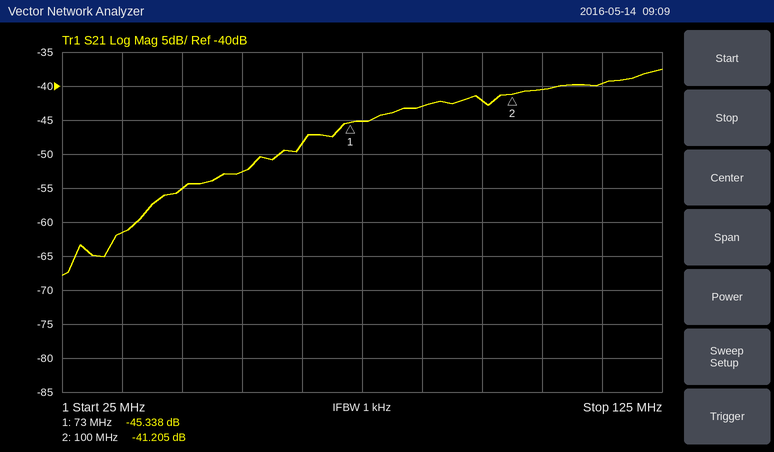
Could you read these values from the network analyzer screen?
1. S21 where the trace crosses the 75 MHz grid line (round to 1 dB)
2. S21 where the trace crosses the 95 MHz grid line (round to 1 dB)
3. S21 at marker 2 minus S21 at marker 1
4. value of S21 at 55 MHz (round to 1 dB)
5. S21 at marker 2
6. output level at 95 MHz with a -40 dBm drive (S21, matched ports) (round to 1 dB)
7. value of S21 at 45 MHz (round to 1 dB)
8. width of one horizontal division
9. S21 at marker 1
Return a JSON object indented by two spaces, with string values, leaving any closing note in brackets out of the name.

{
  "S21 where the trace crosses the 75 MHz grid line": "-45 dB",
  "S21 where the trace crosses the 95 MHz grid line": "-42 dB",
  "S21 at marker 2 minus S21 at marker 1": "4.133 dB",
  "value of S21 at 55 MHz": "-53 dB",
  "S21 at marker 2": "-41.205 dB",
  "output level at 95 MHz with a -40 dBm drive (S21, matched ports)": "-82 dBm",
  "value of S21 at 45 MHz": "-55 dB",
  "width of one horizontal division": "10 MHz",
  "S21 at marker 1": "-45.338 dB"
}
